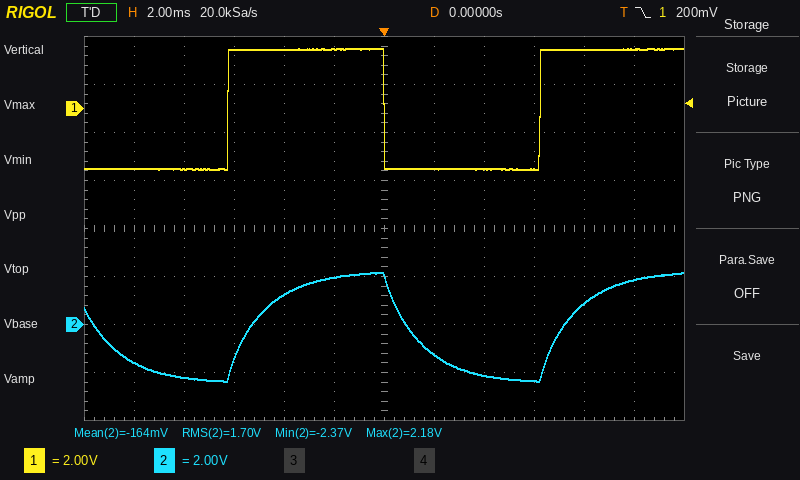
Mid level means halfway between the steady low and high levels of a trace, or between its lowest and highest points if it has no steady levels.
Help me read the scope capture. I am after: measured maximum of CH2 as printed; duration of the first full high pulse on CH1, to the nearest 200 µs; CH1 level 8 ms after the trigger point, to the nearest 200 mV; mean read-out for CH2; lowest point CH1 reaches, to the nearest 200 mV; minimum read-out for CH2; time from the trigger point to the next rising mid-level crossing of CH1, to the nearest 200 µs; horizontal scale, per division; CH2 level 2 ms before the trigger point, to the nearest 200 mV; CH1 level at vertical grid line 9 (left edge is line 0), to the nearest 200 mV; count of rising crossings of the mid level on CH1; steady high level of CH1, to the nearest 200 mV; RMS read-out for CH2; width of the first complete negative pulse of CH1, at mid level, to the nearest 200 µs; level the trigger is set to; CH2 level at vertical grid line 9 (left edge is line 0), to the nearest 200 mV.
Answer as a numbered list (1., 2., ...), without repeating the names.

1. 2.18 V
2. 6.2 ms
3. 2.4 V
4. -164 mV
5. -2.6 V
6. -2.37 V
7. 6.2 ms
8. 2 ms
9. 2.0 V
10. -2.6 V
11. 2
12. 2.4 V
13. 1.70 V
14. 6.2 ms
15. 200 mV
16. -2.4 V
